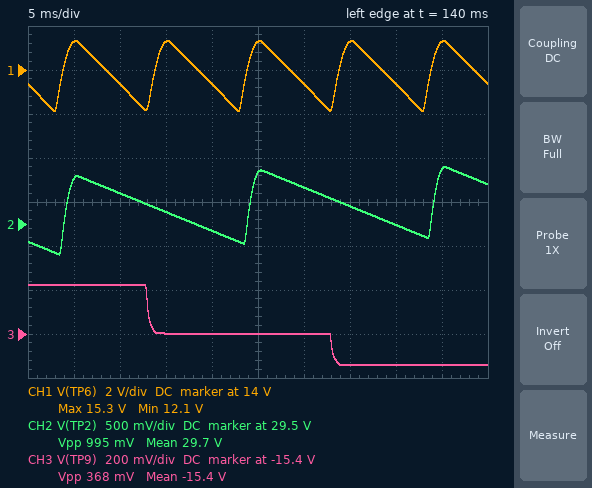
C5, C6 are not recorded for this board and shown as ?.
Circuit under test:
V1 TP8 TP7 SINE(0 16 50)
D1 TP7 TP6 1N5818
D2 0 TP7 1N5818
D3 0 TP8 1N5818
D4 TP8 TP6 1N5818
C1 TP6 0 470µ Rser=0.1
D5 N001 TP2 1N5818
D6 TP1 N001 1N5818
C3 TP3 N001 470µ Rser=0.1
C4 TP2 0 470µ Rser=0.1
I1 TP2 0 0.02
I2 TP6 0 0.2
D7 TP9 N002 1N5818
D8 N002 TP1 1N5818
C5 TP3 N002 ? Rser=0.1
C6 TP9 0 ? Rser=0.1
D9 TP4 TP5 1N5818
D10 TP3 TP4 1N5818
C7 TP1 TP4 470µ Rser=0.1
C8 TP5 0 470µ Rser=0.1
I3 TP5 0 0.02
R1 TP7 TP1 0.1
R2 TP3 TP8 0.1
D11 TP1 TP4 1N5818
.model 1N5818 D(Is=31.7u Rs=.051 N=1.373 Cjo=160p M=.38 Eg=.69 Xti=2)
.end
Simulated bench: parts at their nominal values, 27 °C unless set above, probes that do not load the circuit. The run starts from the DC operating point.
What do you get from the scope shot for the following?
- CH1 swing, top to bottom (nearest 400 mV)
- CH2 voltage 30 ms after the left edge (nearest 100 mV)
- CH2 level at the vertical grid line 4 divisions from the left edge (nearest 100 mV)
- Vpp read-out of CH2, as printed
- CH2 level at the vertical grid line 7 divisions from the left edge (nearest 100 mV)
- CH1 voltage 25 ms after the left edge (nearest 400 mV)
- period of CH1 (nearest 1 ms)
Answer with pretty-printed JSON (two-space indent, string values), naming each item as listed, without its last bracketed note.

{
  "CH1 swing, top to bottom": "3.2 V",
  "CH2 voltage 30 ms after the left edge": "29.9 V",
  "CH2 level at the vertical grid line 4 divisions from the left edge": "29.4 V",
  "Vpp read-out of CH2, as printed": "995 mV",
  "CH2 level at the vertical grid line 7 divisions from the left edge": "29.7 V",
  "CH1 voltage 25 ms after the left edge": "15.2 V",
  "period of CH1": "10 ms"
}
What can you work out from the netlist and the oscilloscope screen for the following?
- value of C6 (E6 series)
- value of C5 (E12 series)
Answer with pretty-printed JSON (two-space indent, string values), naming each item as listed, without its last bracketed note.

{
  "value of C6": "1.5 mF",
  "value of C5": "1 mF"
}
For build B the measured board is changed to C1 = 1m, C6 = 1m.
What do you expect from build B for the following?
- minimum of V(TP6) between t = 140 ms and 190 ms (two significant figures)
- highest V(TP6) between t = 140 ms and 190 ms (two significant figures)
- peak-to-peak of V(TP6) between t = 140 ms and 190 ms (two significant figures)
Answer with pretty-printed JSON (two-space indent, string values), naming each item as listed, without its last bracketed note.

{
  "minimum of V(TP6) between t = 140 ms and 190 ms": "14 V",
  "highest V(TP6) between t = 140 ms and 190 ms": "15 V",
  "peak-to-peak of V(TP6) between t = 140 ms and 190 ms": "1.6 V"
}
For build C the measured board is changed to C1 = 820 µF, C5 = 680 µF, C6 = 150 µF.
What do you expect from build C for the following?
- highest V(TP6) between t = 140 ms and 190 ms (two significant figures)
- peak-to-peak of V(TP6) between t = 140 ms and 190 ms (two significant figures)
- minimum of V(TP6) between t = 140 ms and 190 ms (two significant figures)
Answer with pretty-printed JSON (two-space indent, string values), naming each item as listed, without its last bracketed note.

{
  "highest V(TP6) between t = 140 ms and 190 ms": "15 V",
  "peak-to-peak of V(TP6) between t = 140 ms and 190 ms": "1.9 V",
  "minimum of V(TP6) between t = 140 ms and 190 ms": "13 V"
}
